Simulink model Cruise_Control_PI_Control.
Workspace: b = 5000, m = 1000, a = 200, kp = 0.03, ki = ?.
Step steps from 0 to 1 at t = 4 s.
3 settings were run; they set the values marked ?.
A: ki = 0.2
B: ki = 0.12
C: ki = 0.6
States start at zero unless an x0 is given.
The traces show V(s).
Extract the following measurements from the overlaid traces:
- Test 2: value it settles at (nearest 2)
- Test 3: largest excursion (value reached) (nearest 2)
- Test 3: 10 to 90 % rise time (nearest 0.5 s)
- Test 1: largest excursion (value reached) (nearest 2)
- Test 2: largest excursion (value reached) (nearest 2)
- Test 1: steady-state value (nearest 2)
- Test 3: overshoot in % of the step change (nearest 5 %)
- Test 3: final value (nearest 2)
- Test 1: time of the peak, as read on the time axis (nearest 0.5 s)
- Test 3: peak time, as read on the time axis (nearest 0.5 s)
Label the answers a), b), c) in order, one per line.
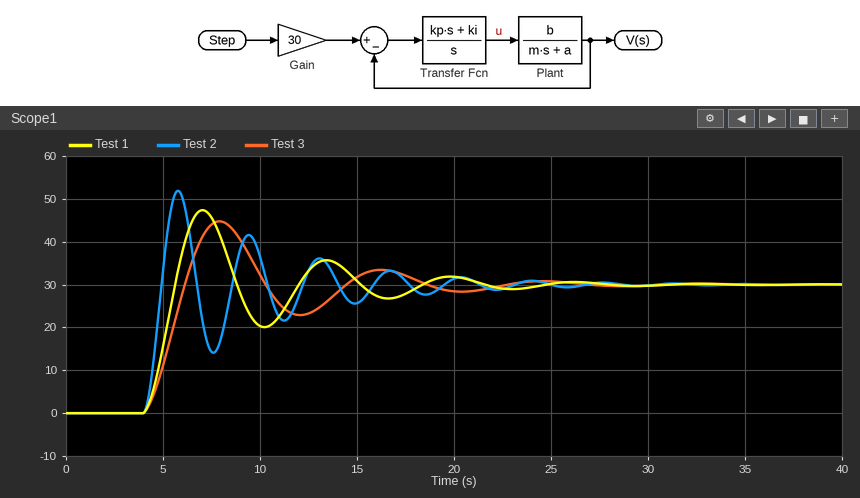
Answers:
a) 30
b) 44
c) 1.5 s
d) 48
e) 52
f) 30
g) 50 %
h) 30
i) 7.0 s
j) 8.0 s
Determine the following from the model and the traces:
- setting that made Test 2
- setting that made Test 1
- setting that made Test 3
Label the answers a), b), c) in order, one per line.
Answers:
a) C
b) A
c) B
